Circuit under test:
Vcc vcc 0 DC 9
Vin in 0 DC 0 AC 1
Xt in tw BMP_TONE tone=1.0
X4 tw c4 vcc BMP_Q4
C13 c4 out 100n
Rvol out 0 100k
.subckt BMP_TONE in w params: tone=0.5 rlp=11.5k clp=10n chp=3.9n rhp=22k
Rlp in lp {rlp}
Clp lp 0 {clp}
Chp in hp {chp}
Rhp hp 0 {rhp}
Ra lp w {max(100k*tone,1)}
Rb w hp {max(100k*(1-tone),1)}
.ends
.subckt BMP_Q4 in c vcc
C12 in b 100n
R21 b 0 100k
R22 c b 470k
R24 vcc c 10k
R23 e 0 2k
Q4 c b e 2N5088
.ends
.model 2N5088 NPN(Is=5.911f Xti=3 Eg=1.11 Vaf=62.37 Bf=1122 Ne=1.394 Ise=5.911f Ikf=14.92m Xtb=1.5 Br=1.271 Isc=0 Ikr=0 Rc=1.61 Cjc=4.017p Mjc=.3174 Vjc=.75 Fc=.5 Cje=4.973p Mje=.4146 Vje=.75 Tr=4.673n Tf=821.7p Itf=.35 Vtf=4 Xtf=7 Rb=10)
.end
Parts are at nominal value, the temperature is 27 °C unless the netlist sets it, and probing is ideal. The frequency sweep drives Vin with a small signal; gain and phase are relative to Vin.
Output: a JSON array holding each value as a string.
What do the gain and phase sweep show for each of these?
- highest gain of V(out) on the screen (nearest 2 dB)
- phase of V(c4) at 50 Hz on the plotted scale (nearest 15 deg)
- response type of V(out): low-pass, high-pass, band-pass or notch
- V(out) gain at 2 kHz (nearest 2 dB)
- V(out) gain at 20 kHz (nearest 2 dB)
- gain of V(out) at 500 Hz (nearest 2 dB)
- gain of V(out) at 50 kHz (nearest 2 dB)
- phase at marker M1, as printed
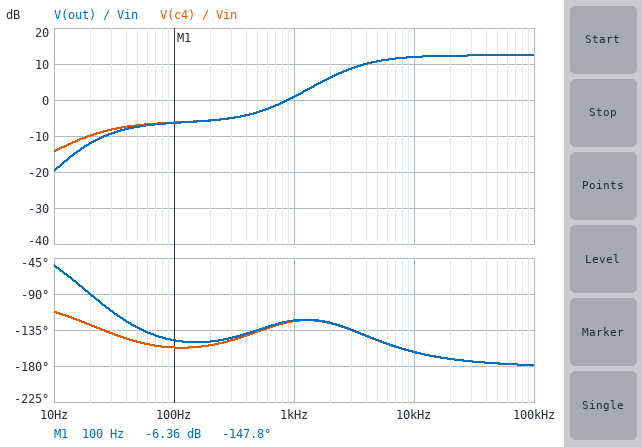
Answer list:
["12 dB", "-150 deg", "high-pass", "6 dB", "12 dB", "-4 dB", "12 dB", "-147.8 deg"]
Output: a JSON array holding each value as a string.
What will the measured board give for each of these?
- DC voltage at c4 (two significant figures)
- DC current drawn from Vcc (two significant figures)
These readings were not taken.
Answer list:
["6.5 V", "250 µA"]
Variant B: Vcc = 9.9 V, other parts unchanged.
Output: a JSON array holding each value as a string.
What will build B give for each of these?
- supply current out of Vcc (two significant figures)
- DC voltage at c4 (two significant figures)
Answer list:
["290 µA", "7.0 V"]
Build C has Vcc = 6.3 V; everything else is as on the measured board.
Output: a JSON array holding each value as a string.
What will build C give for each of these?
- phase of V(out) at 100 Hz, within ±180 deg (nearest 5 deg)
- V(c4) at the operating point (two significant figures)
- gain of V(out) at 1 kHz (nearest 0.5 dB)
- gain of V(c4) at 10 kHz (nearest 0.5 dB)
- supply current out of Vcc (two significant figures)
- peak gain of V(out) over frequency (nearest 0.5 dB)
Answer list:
["-150 deg", "5.0 V", "0.5 dB", "11.5 dB", "130 µA", "12.0 dB"]
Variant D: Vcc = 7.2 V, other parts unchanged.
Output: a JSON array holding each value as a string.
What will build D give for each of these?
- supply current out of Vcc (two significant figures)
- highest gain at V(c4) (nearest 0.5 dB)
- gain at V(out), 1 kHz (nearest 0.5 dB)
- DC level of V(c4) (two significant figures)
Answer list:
["170 µA", "12.0 dB", "0.5 dB", "5.5 V"]
